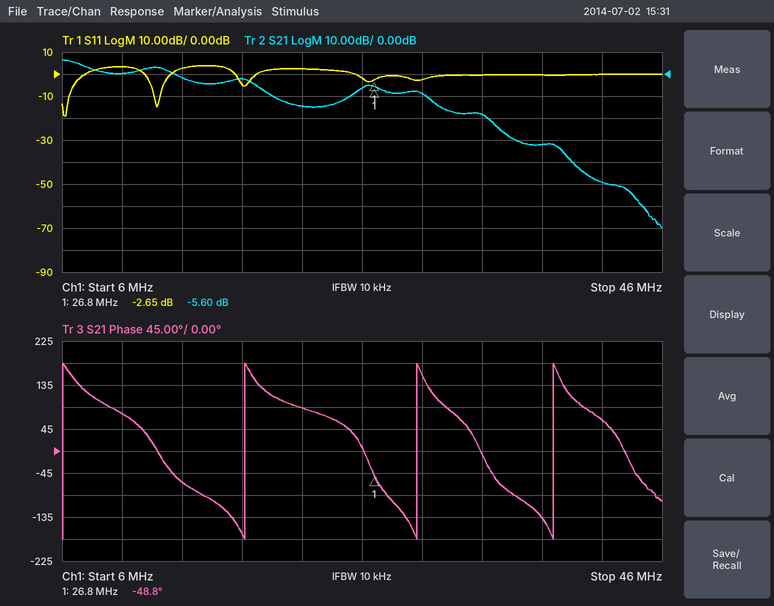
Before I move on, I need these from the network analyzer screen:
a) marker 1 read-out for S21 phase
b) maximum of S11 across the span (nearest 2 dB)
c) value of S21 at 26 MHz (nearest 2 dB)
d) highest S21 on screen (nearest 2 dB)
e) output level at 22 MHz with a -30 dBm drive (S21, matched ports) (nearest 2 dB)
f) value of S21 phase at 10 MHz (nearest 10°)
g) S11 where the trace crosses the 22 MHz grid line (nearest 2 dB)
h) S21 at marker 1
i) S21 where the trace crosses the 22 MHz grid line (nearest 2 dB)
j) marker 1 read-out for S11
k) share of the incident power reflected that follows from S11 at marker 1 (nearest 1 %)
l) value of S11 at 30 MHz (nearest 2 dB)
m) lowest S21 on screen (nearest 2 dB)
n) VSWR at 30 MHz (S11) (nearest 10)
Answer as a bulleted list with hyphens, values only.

- -48.8°
- 4 dB
- -6 dB
- 6 dB
- -44 dBm
- 80°
- 2 dB
- -5.60 dB
- -14 dB
- -2.65 dB
- 54 %
- -2 dB
- -70 dB
- 10
